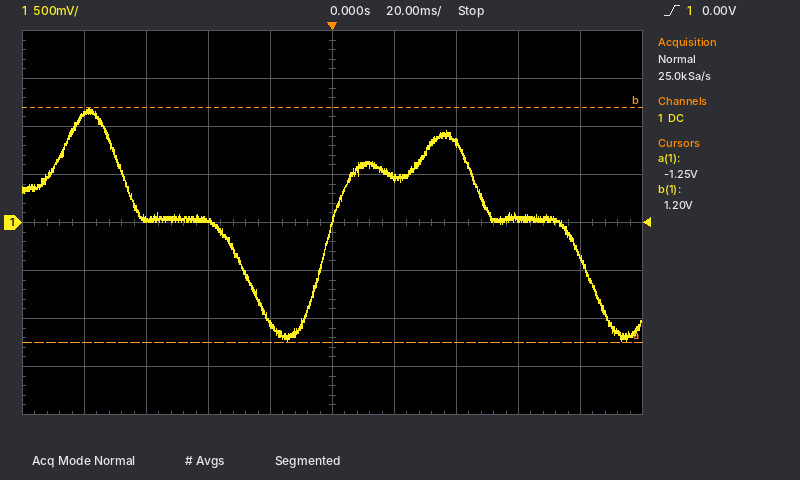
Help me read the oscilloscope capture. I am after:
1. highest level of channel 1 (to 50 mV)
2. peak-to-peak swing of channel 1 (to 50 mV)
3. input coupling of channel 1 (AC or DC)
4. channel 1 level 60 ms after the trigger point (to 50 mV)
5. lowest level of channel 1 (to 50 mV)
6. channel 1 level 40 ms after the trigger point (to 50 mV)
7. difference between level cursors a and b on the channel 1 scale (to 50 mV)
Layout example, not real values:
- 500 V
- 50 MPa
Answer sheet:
- 1.20 V
- 2.45 V
- DC
- 50 mV
- -1.25 V
- 850 mV
- 2.45 V
